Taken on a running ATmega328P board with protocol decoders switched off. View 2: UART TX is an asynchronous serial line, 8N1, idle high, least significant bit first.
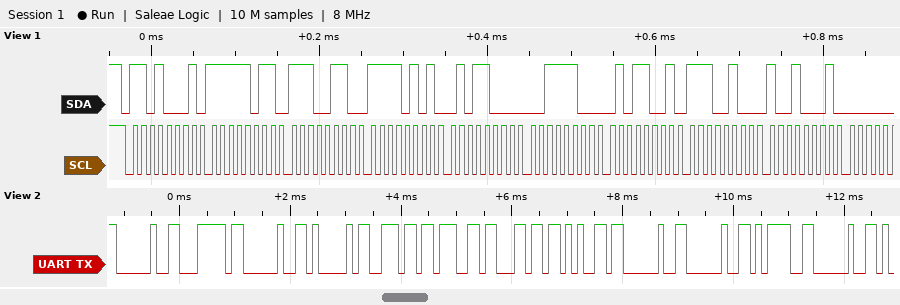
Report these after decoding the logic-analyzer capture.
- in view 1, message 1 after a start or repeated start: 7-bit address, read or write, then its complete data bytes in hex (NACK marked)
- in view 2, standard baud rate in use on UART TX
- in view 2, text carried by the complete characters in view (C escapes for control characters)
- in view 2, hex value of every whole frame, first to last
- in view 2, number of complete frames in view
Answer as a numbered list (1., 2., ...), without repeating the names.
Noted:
1. 0x68 read: FB E6 F5 58 3C 59 E4 91
2. 9600 baud
3. " | Angle  = "
4. 20 7C 20 41 6E 67 6C 65 20 20 3D 20
5. 12
